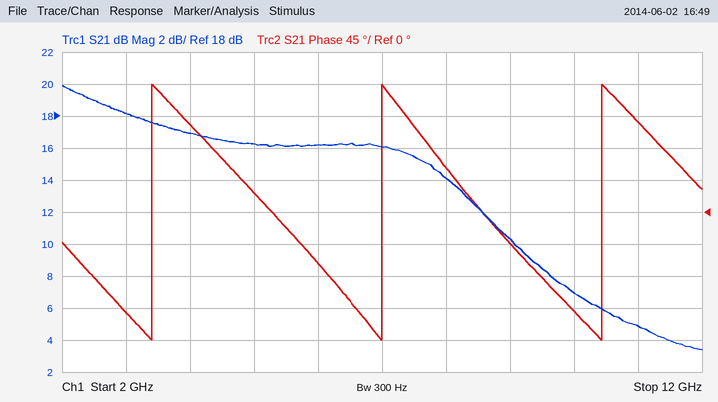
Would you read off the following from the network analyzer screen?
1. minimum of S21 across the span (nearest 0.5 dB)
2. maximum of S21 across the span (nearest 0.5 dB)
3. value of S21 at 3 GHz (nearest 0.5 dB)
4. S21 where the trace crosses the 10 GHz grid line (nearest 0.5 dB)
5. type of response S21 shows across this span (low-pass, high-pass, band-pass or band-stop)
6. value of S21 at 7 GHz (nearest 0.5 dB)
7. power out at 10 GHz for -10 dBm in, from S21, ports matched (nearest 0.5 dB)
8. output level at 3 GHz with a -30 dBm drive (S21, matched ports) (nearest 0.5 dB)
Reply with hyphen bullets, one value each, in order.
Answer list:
- 3.5 dB
- 20.0 dB
- 18.0 dB
- 7.0 dB
- low-pass
- 16.0 dB
- -3.0 dBm
- -12.0 dBm
